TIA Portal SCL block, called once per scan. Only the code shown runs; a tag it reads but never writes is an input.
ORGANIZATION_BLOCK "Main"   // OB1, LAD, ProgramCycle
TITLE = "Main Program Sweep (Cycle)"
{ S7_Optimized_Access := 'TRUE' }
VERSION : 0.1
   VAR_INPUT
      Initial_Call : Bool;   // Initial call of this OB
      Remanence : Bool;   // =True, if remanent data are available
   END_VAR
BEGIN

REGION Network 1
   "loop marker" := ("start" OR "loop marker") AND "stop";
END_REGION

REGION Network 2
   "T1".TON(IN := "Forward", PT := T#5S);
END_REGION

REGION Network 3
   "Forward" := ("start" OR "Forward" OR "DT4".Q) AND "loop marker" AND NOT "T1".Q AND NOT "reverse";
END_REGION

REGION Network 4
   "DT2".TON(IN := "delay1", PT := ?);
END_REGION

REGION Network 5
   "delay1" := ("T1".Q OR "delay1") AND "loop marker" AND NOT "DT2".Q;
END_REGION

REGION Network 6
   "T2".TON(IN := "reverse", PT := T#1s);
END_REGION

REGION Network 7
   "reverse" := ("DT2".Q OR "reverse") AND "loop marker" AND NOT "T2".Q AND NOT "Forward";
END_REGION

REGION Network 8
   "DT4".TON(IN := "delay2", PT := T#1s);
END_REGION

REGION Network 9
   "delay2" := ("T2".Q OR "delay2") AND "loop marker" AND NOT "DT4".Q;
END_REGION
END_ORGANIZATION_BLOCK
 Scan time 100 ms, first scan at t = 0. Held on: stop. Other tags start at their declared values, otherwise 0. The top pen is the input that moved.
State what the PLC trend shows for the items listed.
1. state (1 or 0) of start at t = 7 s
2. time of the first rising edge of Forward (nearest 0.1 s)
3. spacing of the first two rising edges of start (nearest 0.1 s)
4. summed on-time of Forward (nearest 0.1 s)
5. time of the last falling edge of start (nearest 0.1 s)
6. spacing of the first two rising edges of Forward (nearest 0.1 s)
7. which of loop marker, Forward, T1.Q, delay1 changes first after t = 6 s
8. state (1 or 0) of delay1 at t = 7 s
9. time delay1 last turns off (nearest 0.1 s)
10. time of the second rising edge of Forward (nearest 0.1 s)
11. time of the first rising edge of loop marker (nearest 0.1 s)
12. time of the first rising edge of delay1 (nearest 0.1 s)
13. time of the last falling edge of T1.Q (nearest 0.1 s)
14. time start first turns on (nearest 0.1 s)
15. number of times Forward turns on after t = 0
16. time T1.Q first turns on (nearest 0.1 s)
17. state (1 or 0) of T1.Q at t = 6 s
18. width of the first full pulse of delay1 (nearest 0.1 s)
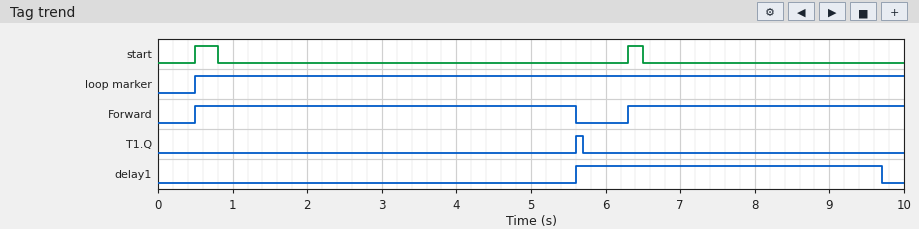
0
0.5 s
5.8 s
8.8 s
6.5 s
5.8 s
Forward
1
9.7 s
6.3 s
0.5 s
5.6 s
5.7 s
0.5 s
2
5.6 s
0
4.1 s
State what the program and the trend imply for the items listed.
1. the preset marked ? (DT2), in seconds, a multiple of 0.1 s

4.0 s
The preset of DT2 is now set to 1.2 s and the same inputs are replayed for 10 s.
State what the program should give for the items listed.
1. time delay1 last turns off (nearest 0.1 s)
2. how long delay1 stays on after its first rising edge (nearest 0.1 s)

6.9 s
1.3 s
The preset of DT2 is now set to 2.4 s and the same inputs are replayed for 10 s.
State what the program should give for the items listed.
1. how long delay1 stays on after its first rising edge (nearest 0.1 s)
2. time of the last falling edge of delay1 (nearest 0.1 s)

2.5 s
8.1 s
